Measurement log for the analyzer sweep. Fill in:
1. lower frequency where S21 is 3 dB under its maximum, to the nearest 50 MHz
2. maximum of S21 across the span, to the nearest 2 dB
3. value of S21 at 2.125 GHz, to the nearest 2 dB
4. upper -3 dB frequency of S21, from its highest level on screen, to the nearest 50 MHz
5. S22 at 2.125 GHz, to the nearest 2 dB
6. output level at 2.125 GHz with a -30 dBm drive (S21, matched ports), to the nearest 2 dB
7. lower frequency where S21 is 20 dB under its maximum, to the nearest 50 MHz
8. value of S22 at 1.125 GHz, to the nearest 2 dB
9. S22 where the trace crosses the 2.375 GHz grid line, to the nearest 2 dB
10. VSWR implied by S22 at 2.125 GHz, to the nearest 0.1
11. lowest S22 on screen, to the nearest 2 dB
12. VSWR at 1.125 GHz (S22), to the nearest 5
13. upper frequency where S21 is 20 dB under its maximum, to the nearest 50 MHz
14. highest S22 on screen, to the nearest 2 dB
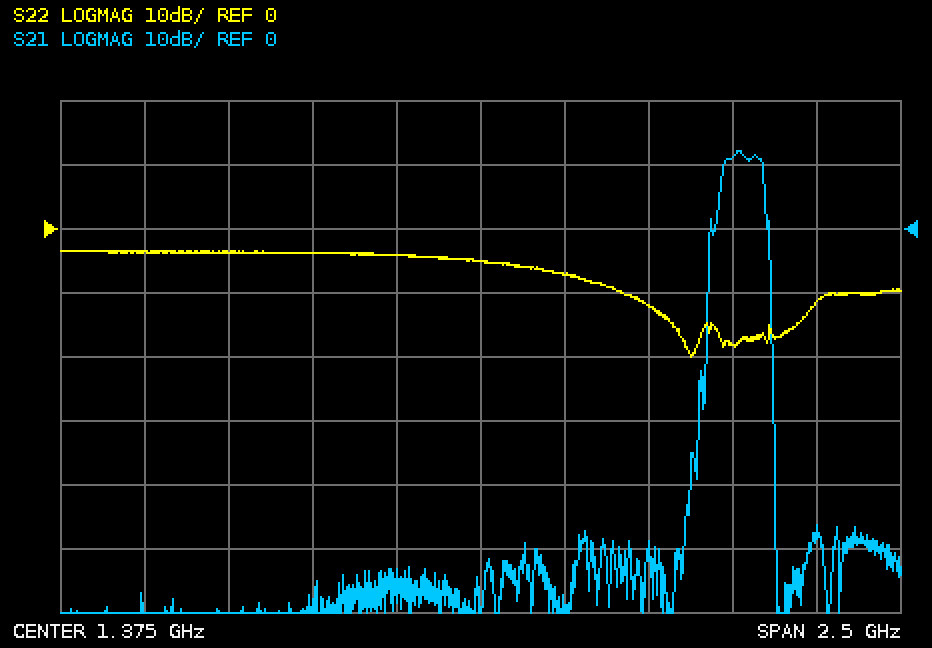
2.10 GHz
12 dB
12 dB
2.20 GHz
-18 dB
-18 dBm
2.05 GHz
-4 dB
-12 dB
1.3
-20 dB
5
2.25 GHz
-4 dB
